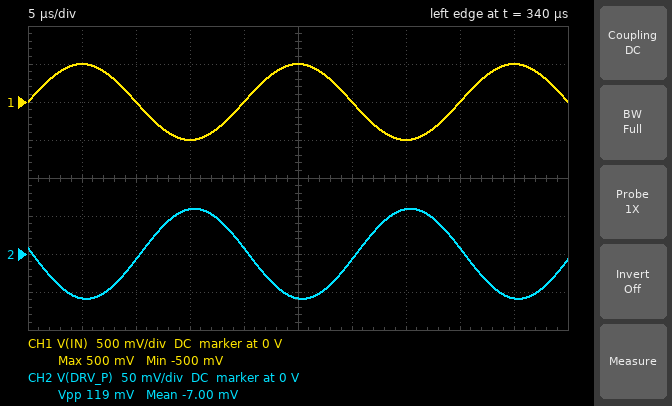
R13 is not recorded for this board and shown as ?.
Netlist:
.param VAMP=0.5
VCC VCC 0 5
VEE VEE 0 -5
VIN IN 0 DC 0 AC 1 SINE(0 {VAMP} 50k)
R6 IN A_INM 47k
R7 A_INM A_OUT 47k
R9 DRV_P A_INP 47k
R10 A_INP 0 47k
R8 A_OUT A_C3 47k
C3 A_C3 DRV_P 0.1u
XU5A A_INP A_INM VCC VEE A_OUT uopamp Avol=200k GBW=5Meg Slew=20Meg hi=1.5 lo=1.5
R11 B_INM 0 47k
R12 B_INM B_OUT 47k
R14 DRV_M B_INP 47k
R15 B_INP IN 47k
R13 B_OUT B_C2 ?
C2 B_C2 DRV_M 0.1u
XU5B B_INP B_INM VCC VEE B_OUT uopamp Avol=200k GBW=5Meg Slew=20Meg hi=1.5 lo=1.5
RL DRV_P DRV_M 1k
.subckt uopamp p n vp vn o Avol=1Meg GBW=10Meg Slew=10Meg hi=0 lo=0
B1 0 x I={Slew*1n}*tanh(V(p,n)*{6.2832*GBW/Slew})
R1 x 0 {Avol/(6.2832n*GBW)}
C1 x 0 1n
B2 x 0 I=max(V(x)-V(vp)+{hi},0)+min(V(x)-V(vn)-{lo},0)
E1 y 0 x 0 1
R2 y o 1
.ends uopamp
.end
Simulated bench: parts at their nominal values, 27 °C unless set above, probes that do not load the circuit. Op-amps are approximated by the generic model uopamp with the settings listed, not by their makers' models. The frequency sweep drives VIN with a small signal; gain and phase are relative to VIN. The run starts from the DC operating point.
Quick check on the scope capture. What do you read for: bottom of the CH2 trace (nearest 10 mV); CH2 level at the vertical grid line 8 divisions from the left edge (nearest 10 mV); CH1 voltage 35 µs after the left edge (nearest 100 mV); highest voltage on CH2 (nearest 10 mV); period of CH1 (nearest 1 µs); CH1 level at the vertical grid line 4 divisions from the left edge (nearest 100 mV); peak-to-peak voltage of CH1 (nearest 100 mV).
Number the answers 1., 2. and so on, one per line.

1. -60 mV
2. 10 mV
3. -500 mV
4. 60 mV
5. 20 µs
6. 0 V
7. 1.0 V
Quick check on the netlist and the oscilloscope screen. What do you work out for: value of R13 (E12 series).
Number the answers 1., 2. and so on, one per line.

1. 120 kΩ
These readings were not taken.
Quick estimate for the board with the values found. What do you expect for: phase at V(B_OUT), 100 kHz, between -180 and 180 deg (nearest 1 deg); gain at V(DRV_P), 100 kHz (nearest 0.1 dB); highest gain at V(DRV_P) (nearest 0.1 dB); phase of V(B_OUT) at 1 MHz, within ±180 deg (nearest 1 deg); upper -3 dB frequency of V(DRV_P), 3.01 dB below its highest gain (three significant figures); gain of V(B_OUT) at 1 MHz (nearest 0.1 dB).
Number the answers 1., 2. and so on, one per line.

1. 0 deg
2. -18.5 dB
3. -4.7 dB
4. -13 deg
5. 49.7 Hz
6. -0.1 dB
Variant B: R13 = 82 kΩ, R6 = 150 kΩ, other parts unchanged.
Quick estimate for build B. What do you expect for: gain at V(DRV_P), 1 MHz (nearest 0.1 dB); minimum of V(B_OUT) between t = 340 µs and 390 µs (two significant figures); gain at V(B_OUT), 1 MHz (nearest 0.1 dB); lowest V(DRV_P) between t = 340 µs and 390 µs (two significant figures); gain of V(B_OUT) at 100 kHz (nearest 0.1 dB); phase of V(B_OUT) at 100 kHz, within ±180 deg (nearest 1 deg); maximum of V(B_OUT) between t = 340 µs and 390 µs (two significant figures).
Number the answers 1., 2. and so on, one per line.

1. -6.6 dB
2. -790 mV
3. 2.6 dB
4. -280 mV
5. 3.9 dB
6. -3 deg
7. 790 mV
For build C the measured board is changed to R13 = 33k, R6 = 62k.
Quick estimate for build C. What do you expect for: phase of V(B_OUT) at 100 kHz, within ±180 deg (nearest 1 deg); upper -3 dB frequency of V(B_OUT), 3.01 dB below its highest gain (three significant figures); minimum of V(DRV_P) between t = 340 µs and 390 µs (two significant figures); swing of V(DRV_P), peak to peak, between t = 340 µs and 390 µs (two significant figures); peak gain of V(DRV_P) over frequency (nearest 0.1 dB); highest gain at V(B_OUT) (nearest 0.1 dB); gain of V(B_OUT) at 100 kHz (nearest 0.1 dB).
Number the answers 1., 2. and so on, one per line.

1. -5 deg
2. 1.02 MHz
3. -510 mV
4. 1.0 V
5. 0.2 dB
6. 6.3 dB
7. 6.2 dB
